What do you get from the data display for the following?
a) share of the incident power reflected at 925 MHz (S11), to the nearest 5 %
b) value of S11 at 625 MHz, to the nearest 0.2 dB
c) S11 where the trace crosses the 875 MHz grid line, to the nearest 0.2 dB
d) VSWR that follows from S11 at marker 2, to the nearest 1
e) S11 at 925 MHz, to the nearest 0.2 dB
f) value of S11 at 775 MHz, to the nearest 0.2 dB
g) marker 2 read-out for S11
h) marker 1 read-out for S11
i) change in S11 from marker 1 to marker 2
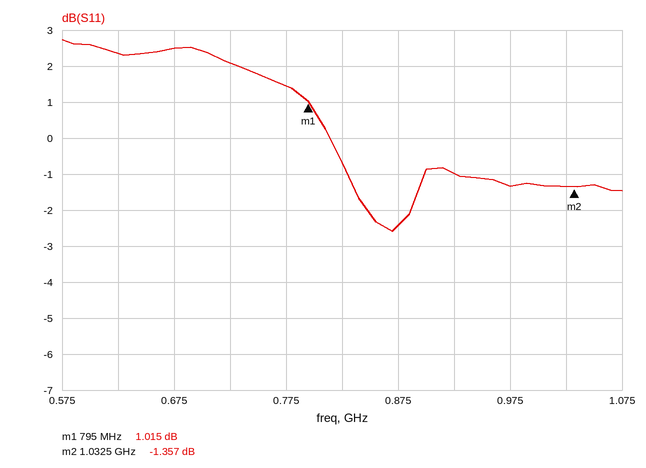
80 %
2.4 dB
-2.4 dB
13
-1.0 dB
1.4 dB
-1.357 dB
1.015 dB
-2.372 dB
